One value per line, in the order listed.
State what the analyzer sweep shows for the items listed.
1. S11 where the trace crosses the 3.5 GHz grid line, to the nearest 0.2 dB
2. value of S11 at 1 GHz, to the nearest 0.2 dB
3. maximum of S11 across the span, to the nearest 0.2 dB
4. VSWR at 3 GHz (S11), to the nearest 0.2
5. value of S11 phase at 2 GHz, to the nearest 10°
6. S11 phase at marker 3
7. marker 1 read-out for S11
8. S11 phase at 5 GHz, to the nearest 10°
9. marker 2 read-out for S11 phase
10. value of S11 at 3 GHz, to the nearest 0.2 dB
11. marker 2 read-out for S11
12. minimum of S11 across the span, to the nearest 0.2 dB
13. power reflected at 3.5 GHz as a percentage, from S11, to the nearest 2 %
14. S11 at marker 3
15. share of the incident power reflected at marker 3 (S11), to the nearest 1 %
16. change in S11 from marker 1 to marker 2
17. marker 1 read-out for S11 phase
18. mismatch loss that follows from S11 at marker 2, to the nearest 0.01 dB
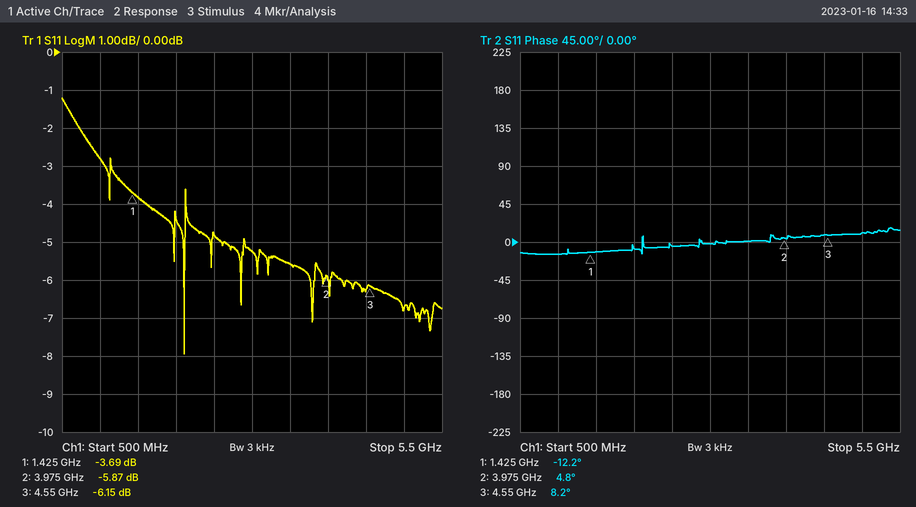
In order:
-5.6 dB
-2.8 dB
-1.2 dB
3.4
-10°
8.2°
-3.69 dB
10°
4.8°
-5.2 dB
-5.87 dB
-8.0 dB
28 %
-6.15 dB
24 %
-2.18 dB
-12.2°
1.30 dB
